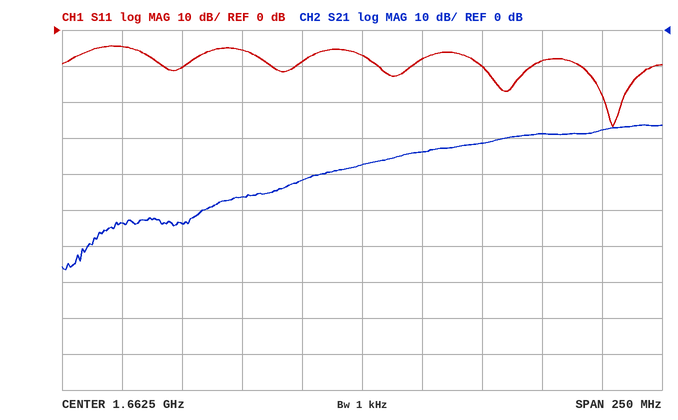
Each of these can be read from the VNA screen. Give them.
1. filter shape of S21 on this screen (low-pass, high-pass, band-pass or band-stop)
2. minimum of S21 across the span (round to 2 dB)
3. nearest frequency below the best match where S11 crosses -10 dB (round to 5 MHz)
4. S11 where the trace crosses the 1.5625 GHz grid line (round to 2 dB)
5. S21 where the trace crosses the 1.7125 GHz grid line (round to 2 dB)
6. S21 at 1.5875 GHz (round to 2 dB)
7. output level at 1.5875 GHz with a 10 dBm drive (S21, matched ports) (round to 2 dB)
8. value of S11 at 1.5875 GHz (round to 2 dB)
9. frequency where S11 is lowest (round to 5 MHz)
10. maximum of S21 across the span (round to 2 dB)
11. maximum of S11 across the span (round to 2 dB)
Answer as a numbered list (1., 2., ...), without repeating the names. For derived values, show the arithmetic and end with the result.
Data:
1. high-pass
2. -66 dB
3. 1.755 GHz
4. -4 dB
5. -32 dB
6. -54 dB
7. 10 dBm + (-54 dB) = -44 dBm
8. -10 dB
9. 1.765 GHz
10. -26 dB
11. -4 dB
